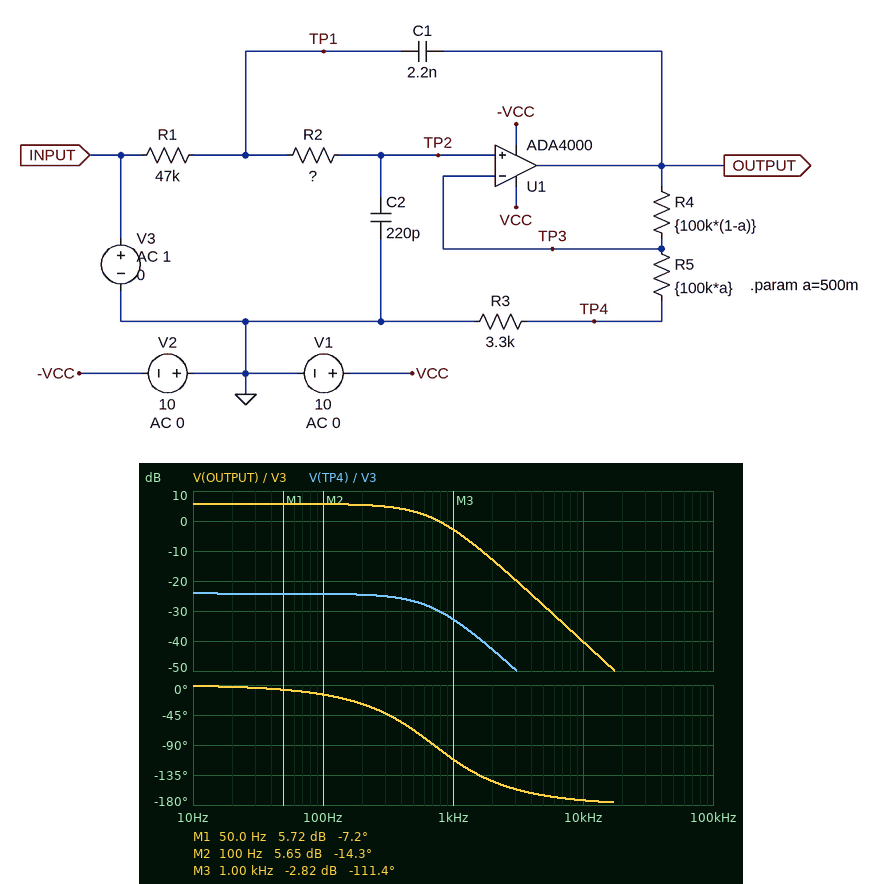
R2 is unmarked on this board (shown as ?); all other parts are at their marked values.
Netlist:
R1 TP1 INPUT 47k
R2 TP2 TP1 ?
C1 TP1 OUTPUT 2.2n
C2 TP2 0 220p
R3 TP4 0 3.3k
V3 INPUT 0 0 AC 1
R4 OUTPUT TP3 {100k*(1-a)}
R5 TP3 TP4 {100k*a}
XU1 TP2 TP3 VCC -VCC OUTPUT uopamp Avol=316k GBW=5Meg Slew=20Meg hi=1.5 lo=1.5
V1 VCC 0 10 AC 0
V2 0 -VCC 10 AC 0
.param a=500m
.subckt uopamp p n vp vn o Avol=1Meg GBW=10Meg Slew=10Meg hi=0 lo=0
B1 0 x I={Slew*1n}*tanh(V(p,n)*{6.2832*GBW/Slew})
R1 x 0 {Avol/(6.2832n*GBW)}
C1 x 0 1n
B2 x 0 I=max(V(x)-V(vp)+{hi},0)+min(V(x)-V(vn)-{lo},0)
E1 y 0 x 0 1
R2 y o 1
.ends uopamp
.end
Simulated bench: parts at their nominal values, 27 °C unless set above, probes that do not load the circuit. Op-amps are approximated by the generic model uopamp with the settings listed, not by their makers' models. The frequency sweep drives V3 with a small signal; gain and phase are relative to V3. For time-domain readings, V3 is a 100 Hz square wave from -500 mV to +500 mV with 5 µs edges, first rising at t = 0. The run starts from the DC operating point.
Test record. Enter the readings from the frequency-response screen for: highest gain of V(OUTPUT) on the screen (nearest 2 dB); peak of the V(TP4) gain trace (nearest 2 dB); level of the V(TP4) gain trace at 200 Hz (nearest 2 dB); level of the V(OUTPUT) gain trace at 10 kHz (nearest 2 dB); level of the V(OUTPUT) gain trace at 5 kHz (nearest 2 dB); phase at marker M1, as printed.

6 dB
-24 dB
-24 dB
-40 dB
-28 dB
-7.2 deg
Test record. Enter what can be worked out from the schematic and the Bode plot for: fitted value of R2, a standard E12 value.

2.2 MΩ
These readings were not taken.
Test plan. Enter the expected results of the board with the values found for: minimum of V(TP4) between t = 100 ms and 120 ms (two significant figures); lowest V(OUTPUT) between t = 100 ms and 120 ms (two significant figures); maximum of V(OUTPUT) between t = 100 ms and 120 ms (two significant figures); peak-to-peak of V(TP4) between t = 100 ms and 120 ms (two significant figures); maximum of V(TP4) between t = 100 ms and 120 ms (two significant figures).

-31 mV
-970 mV
970 mV
62 mV
31 mV
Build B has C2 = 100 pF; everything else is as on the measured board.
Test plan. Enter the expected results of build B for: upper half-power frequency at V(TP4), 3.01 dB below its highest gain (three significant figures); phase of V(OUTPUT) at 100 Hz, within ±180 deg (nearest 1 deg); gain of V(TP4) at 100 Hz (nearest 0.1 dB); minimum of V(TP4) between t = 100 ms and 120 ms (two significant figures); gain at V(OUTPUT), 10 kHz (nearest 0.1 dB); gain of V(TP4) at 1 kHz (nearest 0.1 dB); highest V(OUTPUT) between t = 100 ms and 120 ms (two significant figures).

1.25 kHz
-5 deg
-24.1 dB
-45 mV
-33.3 dB
-22.3 dB
1.4 V
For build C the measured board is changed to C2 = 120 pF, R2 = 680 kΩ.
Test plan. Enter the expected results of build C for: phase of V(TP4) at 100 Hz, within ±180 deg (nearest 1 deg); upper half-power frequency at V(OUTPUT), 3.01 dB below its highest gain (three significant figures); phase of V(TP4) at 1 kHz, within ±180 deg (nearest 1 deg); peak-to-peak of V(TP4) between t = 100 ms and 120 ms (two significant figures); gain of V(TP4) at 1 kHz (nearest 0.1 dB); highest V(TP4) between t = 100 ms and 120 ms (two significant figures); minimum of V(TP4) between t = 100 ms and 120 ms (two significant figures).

0 deg
1.82 kHz
5 deg
540 mV
-20.7 dB
270 mV
-270 mV
